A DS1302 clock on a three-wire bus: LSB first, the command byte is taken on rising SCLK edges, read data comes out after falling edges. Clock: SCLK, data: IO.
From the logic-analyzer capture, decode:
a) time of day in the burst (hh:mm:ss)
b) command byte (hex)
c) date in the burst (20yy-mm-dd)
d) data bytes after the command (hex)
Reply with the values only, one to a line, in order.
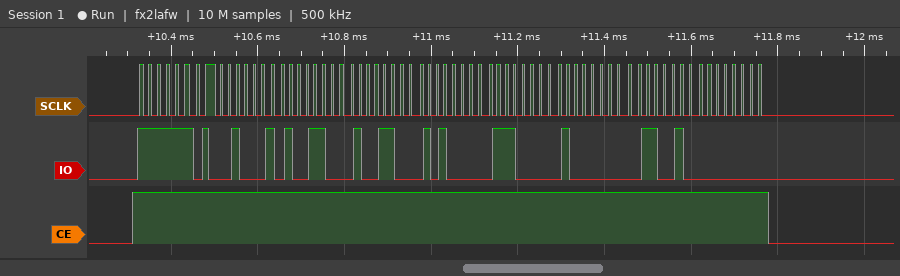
19:19:44
0xBF
2026-07-05
44 19 19 05 07 01 26 00
